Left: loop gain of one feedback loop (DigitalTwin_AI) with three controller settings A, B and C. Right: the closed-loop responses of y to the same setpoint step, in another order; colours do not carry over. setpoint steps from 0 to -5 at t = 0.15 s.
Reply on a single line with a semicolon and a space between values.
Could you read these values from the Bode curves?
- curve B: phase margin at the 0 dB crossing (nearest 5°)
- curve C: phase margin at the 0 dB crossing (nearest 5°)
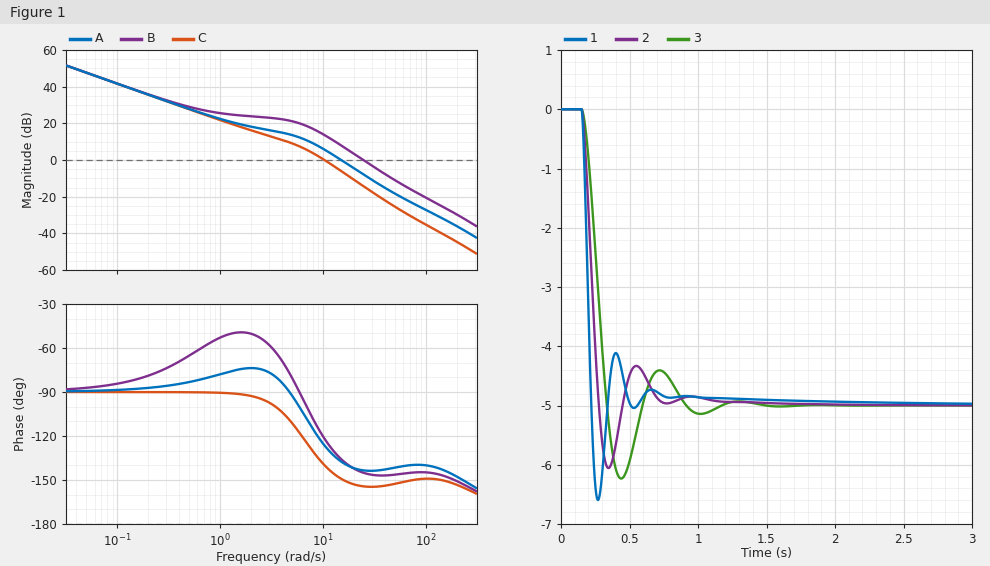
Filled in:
35°; 40°
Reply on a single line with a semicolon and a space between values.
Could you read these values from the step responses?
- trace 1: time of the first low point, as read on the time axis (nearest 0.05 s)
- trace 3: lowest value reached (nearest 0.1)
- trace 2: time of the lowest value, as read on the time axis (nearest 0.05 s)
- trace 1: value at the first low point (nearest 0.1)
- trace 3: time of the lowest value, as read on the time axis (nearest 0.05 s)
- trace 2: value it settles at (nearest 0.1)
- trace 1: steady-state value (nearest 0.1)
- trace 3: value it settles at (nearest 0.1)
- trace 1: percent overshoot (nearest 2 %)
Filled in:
0.25 s; -6.2; 0.35 s; -6.6; 0.45 s; -5.0; -5.0; -5.0; 32 %
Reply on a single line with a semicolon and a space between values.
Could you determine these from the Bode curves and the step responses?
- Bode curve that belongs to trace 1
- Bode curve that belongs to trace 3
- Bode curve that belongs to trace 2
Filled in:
B; C; A
